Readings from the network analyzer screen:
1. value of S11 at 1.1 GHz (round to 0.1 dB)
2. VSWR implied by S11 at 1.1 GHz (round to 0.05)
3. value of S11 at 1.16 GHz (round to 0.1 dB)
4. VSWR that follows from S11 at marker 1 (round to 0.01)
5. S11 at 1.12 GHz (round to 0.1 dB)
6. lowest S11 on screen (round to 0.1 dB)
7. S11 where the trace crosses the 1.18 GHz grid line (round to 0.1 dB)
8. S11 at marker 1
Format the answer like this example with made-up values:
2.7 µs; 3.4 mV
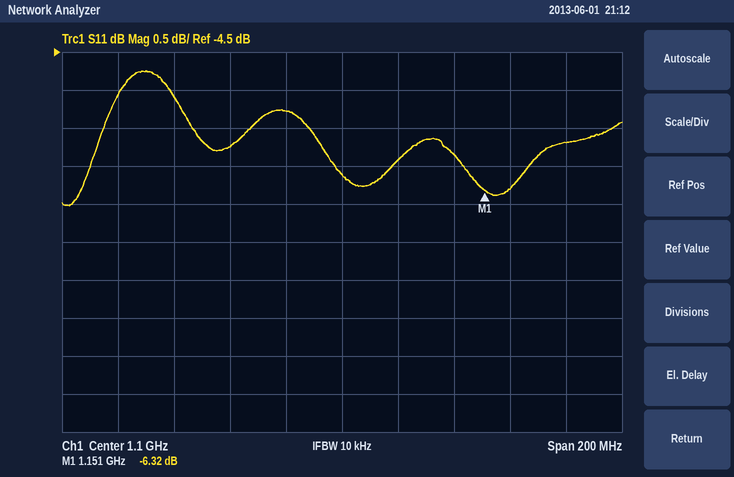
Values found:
-6.1 dB; 2.95; -6.3 dB; 2.87; -5.9 dB; -6.5 dB; -5.7 dB; -6.32 dB
